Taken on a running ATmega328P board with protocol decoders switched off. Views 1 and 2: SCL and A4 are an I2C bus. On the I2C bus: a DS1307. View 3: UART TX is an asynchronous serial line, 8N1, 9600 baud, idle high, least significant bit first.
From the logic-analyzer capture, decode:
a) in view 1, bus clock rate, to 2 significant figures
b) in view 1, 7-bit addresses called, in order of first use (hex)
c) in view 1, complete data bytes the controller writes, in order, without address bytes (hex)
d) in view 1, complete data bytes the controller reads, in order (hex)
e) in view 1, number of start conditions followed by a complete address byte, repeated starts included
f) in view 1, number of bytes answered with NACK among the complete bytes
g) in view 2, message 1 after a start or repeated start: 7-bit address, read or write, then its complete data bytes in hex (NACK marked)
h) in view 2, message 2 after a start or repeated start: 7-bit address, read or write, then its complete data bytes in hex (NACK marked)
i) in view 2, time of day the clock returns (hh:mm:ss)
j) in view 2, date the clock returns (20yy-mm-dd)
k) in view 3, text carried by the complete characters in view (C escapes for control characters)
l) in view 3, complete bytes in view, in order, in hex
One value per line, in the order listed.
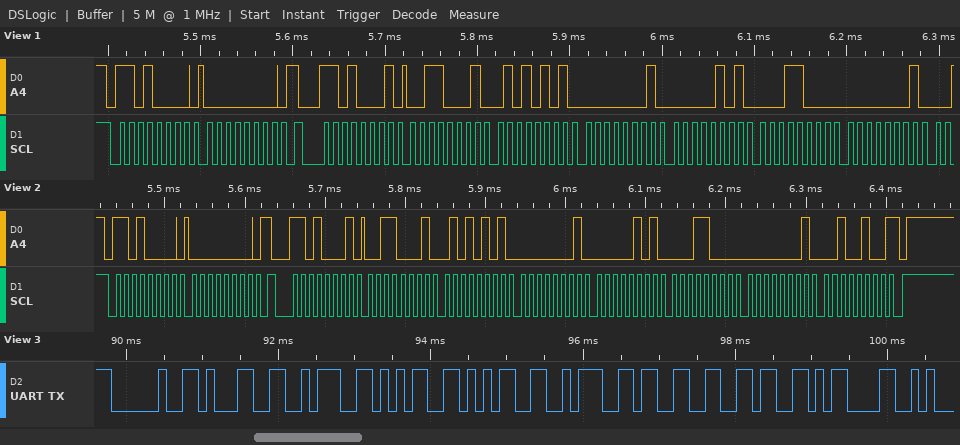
100 kHz
0x68
00
31 55 01 05 18 01
2
0
0x68 write: 00
0x68 read: 31 55 01 05 18 01 24 NACK
01:55:31
2024-01-18
" 1:55:36\r"
20 31 3A 35 35 3A 33 36 0D
